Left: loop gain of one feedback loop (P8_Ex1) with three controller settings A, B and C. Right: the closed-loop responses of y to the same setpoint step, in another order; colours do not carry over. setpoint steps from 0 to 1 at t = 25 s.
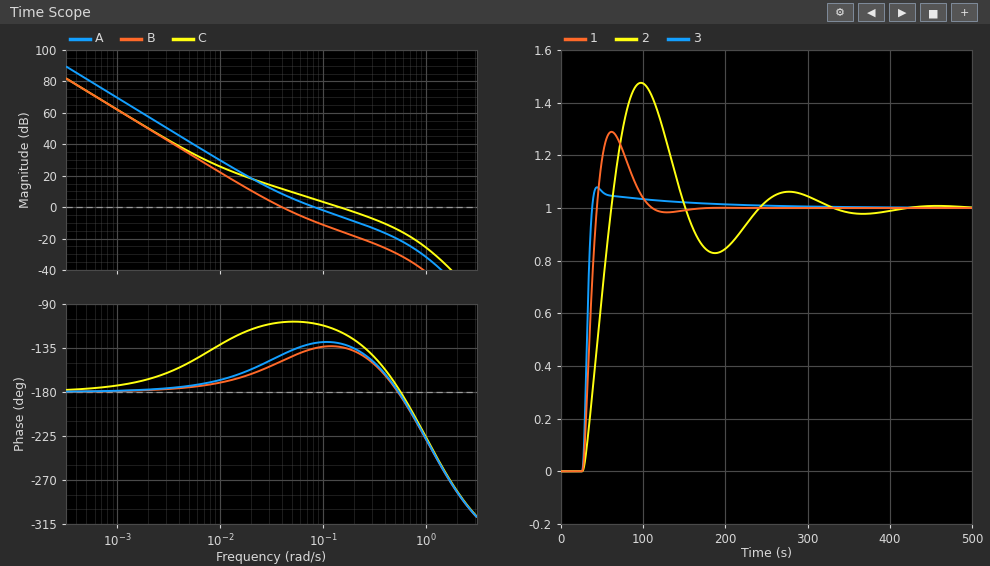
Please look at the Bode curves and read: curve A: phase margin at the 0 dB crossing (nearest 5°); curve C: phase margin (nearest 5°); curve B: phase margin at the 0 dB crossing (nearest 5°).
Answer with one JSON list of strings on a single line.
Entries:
["50°", "60°", "30°"]
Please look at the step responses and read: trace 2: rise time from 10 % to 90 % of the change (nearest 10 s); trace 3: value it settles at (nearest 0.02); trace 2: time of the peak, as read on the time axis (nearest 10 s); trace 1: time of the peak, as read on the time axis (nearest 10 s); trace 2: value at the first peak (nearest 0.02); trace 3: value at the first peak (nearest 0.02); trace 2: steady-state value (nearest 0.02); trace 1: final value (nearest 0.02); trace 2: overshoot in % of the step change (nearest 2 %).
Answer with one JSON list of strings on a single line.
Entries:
["30 s", "1.00", "100 s", "60 s", "1.48", "1.08", "1.00", "1.00", "48 %"]
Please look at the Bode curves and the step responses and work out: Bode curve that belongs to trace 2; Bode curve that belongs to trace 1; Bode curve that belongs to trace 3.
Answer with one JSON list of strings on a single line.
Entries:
["B", "A", "C"]
